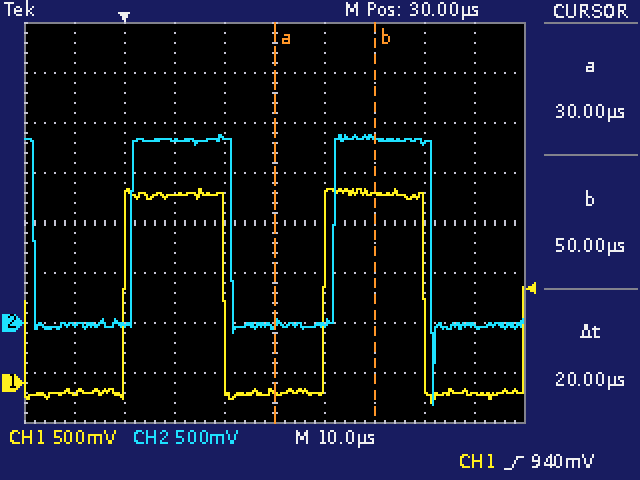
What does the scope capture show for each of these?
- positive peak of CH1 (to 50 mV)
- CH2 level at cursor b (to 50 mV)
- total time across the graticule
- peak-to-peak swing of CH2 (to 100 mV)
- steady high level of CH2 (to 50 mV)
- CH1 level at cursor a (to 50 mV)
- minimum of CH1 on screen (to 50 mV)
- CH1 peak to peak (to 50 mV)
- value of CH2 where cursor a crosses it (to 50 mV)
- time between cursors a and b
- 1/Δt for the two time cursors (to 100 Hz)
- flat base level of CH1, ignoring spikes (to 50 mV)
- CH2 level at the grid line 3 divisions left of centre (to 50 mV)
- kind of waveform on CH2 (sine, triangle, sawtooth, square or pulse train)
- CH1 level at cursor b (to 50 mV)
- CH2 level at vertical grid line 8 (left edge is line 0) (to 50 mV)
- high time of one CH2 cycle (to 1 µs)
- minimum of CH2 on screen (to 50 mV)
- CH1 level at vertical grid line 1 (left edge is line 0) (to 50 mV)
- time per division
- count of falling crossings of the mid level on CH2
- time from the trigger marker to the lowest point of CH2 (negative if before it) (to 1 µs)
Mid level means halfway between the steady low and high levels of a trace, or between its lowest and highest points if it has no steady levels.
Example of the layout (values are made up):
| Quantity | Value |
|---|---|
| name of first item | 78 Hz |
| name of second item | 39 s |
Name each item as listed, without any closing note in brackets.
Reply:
| Quantity | Value |
|---|---|
| positive peak of CH1 | 1.95 V |
| CH2 level at cursor b | 1.85 V |
| total time across the graticule | 100 µs |
| peak-to-peak swing of CH2 | 2.70 V |
| steady high level of CH2 | 1.85 V |
| CH1 level at cursor a | -100 mV |
| minimum of CH1 on screen | -200 mV |
| CH1 peak to peak | 2.15 V |
| value of CH2 where cursor a crosses it | 0 mV |
| time between cursors a and b | 20 µs |
| 1/Δt for the two time cursors | 50.0 kHz |
| flat base level of CH1, ignoring spikes | -100 mV |
| CH2 level at the grid line 3 divisions left of centre | 0 mV |
| kind of waveform on CH2 | square |
| CH1 level at cursor b | 1.90 V |
| CH2 level at vertical grid line 8 (left edge is line 0) | 1.80 V |
| high time of one CH2 cycle | 20 µs |
| minimum of CH2 on screen | -800 mV |
| CH1 level at vertical grid line 1 (left edge is line 0) | -100 mV |
| time per division | 10 µs |
| count of falling crossings of the mid level on CH2 | 3 |
| time from the trigger marker to the lowest point of CH2 (negative if before it) | +62 µs |
